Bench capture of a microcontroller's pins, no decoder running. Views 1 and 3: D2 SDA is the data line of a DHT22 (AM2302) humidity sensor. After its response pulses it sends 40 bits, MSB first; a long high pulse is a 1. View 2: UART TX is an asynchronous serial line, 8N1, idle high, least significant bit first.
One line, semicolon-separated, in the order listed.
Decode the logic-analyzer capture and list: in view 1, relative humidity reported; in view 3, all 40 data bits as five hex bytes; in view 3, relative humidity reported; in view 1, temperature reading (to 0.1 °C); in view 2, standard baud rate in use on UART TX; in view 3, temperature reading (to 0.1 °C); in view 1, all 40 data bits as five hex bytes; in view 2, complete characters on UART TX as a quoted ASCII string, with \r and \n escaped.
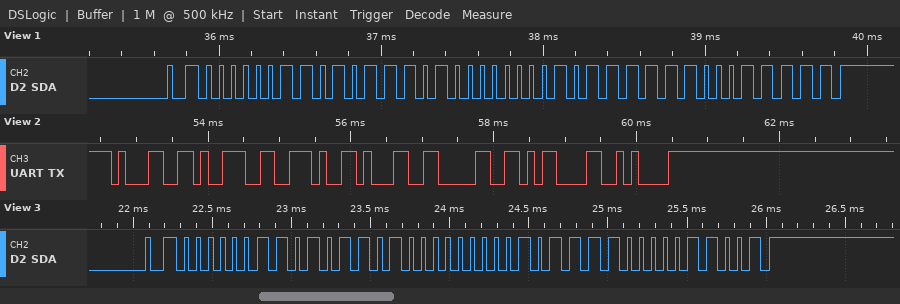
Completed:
86.1 %; 03 5A 00 BC 19; 85.8 %; 19.1 °C; 9600 baud; 18.8 °C; 03 5D 00 BF 1F; "19.10\r\n"
